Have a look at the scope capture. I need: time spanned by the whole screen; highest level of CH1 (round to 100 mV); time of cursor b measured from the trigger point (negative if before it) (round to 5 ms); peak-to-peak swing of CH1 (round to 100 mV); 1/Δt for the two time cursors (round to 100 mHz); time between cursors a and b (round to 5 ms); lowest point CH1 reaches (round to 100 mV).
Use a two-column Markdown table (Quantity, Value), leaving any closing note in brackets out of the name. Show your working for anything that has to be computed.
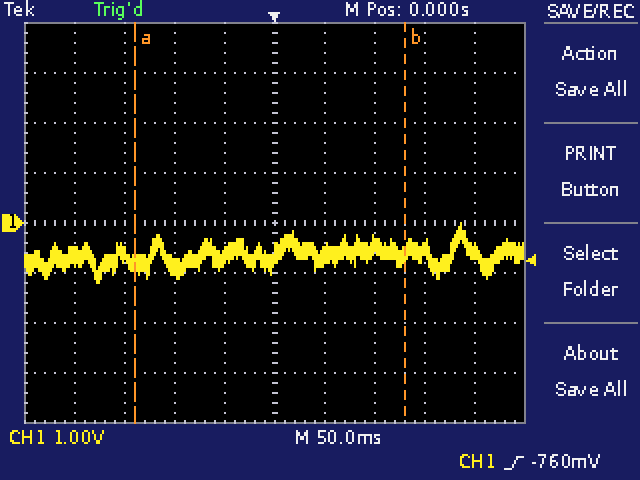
| Quantity | Value |
|---|---|
| time spanned by the whole screen | 500 ms |
| highest level of CH1 | 0.0 V |
| time of cursor b measured from the trigger point (negative if before it) | +130 ms |
| peak-to-peak swing of CH1 | 0.0 V − (-1.2 V) = 1.2 V |
| 1/Δt for the two time cursors | 1 / 270 ms ≈ 3.7 Hz |
| time between cursors a and b | 270 ms |
| lowest point CH1 reaches | -1.2 V |
